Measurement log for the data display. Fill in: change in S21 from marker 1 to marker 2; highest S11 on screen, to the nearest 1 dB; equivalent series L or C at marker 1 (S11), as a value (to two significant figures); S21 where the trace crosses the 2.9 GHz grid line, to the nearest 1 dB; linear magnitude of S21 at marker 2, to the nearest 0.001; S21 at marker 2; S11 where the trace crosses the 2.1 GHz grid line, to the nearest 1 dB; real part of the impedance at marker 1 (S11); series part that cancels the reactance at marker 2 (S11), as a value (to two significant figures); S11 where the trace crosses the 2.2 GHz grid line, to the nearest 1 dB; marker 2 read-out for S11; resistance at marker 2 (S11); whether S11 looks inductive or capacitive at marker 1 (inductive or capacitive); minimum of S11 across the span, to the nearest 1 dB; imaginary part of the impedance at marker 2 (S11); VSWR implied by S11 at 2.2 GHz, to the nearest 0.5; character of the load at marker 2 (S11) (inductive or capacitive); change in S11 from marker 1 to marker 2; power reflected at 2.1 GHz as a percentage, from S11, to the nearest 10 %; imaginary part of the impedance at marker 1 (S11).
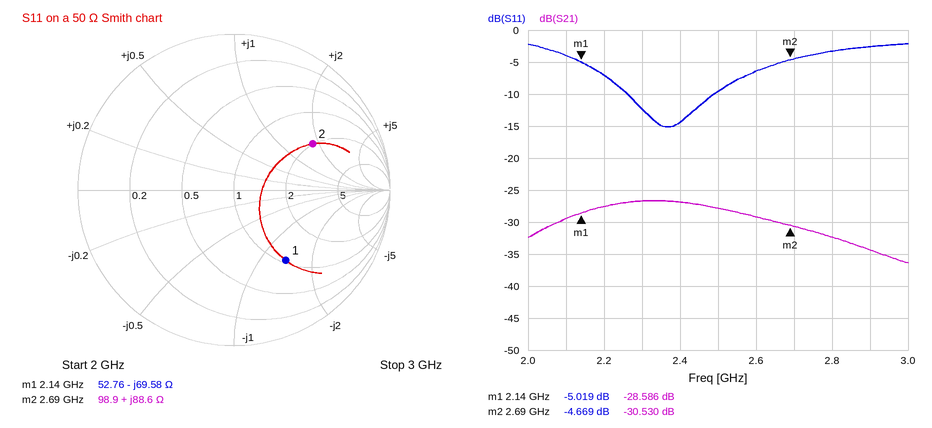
-1.944 dB
-2 dB
1.1 pF
-34 dB
0.030
-30.530 dB
-4 dB
52.76 Ω
670 fF
-7 dB
-4.669 dB
98.9 Ω
capacitive
-15 dB
+88.6 Ω
2.5
inductive
0.350 dB
40 %
-69.58 Ω
